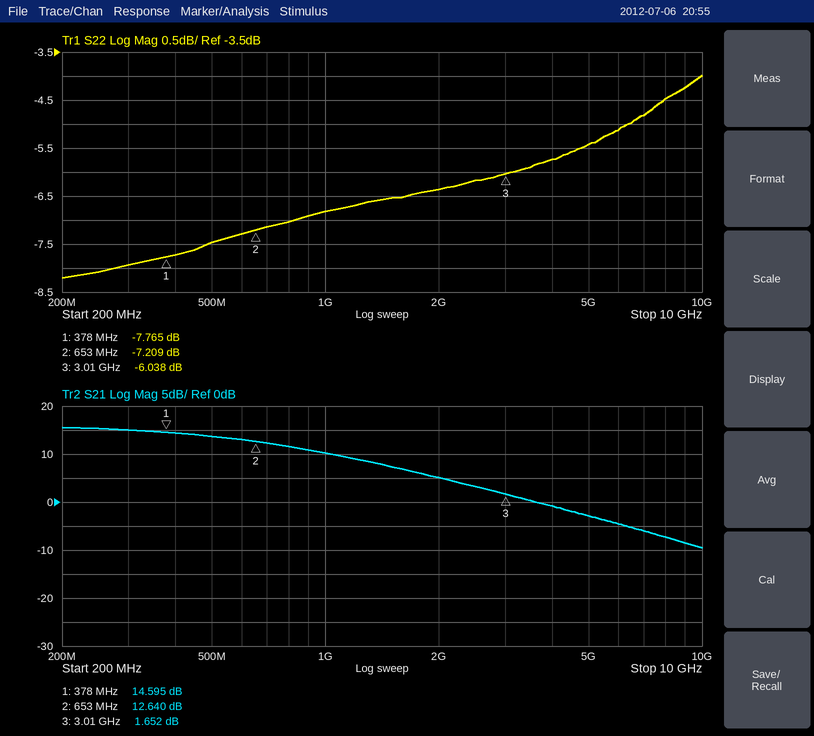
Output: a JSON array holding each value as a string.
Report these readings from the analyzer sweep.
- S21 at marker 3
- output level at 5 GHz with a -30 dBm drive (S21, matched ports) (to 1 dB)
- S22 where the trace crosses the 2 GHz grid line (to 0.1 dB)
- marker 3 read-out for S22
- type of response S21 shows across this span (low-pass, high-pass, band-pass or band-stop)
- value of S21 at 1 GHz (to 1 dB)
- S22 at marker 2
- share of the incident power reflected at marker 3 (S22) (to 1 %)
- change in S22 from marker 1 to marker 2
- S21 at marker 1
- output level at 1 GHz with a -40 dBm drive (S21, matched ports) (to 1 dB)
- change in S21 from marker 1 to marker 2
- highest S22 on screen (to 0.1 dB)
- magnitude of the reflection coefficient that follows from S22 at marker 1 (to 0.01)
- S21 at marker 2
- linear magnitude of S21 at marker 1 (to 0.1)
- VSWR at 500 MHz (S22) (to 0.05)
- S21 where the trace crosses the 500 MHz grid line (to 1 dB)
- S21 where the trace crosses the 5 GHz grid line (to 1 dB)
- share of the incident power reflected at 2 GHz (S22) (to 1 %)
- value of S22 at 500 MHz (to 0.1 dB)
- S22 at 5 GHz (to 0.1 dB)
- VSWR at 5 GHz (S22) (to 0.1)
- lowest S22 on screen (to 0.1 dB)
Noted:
["1.652 dB", "-33 dBm", "-6.4 dB", "-6.038 dB", "low-pass", "10 dB", "-7.209 dB", "25 %", "0.556 dB", "14.595 dB", "-30 dBm", "-1.955 dB", "-4.0 dB", "0.41", "12.640 dB", "5.4", "2.45", "14 dB", "-3 dB", "23 %", "-7.5 dB", "-5.4 dB", "3.3", "-8.2 dB"]
